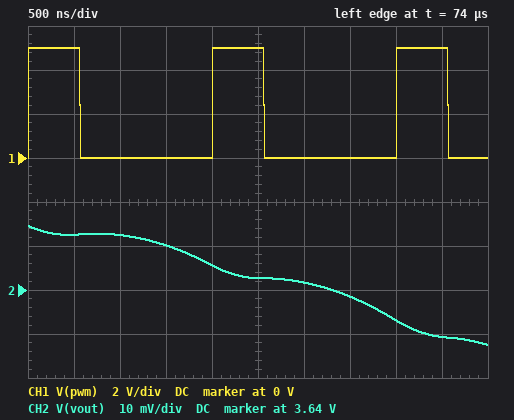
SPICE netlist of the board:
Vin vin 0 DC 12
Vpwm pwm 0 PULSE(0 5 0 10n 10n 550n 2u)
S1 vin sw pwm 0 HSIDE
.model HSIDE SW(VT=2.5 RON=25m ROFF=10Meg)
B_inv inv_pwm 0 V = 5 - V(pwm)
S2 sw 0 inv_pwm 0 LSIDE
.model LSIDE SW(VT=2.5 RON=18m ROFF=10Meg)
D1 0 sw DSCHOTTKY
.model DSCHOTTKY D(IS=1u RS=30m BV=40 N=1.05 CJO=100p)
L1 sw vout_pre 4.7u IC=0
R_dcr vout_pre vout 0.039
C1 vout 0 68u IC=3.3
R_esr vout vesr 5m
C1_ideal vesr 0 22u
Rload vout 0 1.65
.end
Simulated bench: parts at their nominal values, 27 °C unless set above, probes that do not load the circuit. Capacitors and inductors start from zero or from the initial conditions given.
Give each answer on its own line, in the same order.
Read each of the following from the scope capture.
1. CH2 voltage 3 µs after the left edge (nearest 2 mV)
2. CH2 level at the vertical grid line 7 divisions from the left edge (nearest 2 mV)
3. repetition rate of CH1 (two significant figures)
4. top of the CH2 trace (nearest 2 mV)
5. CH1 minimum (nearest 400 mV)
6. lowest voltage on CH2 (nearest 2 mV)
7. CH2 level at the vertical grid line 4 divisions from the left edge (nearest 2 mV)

3.642 V
3.638 V
500 kHz
3.654 V
0 V
3.628 V
3.646 V
